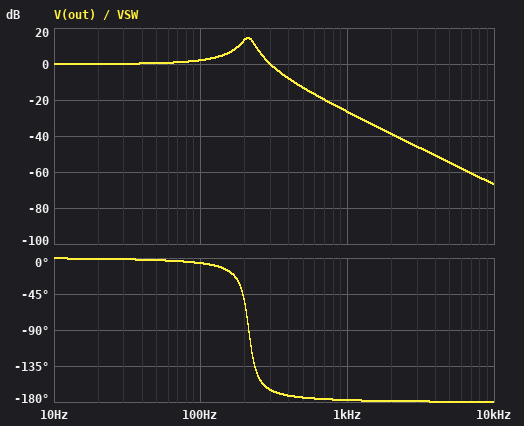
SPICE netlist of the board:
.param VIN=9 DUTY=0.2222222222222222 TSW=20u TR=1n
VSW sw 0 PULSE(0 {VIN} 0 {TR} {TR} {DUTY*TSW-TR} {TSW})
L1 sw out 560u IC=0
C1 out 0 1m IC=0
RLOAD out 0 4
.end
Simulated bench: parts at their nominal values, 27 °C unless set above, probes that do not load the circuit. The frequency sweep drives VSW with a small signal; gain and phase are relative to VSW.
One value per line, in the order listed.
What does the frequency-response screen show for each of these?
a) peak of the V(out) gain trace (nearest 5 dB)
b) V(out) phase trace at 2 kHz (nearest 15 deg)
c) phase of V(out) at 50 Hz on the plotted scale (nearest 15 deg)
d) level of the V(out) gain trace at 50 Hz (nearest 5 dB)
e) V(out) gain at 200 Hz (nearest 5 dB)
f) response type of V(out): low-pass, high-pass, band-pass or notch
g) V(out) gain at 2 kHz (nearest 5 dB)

15 dB
-180 deg
0 deg
0 dB
15 dB
low-pass
-40 dB
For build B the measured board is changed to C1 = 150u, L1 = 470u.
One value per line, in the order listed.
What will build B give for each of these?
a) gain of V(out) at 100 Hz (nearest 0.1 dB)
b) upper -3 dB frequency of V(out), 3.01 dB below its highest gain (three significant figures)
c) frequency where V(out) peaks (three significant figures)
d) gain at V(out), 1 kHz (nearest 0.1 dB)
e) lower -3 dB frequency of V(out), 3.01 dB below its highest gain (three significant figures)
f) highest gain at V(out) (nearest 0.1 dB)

0.2 dB
692 Hz
569 Hz
-5.7 dB
411 Hz
7.3 dB
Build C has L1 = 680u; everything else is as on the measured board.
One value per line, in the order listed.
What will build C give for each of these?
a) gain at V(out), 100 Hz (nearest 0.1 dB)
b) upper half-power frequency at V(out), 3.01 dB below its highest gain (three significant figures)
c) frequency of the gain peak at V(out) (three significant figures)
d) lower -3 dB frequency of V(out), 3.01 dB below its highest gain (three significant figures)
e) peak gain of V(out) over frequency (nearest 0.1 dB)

2.6 dB
210 Hz
191 Hz
170 Hz
13.8 dB
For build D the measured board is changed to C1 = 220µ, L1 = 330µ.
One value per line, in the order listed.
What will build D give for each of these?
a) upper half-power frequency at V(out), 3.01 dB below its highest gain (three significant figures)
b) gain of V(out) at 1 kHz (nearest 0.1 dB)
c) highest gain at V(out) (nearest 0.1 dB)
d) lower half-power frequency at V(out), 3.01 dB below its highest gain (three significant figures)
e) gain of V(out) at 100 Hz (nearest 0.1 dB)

662 Hz
-5.7 dB
10.4 dB
476 Hz
0.2 dB
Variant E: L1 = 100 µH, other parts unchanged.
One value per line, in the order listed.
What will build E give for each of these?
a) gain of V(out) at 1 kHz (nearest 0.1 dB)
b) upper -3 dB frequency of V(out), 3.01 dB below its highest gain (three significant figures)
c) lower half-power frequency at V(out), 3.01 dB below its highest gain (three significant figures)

-9.4 dB
522 Hz
482 Hz
